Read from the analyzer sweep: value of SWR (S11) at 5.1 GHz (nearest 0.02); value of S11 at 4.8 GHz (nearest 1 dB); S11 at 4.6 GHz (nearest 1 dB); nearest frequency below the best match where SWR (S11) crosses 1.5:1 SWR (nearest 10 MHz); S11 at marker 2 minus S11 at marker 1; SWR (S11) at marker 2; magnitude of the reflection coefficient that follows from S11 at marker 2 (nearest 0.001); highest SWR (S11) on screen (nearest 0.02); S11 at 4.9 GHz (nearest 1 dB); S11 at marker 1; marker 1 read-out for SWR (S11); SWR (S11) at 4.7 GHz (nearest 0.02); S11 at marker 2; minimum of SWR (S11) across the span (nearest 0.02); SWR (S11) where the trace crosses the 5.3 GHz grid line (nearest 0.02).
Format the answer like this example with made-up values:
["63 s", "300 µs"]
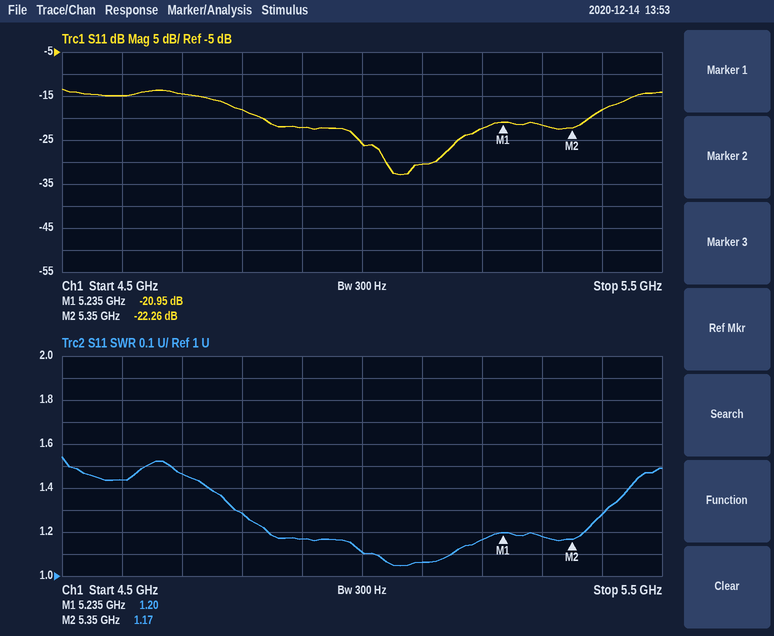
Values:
["1.06", "-18 dB", "-15 dB", "4.68 GHz", "-1.31 dB", "1.17", "0.077", "1.54", "-22 dB", "-20.95 dB", "1.20", "1.46", "-22.26 dB", "1.04", "1.18"]
